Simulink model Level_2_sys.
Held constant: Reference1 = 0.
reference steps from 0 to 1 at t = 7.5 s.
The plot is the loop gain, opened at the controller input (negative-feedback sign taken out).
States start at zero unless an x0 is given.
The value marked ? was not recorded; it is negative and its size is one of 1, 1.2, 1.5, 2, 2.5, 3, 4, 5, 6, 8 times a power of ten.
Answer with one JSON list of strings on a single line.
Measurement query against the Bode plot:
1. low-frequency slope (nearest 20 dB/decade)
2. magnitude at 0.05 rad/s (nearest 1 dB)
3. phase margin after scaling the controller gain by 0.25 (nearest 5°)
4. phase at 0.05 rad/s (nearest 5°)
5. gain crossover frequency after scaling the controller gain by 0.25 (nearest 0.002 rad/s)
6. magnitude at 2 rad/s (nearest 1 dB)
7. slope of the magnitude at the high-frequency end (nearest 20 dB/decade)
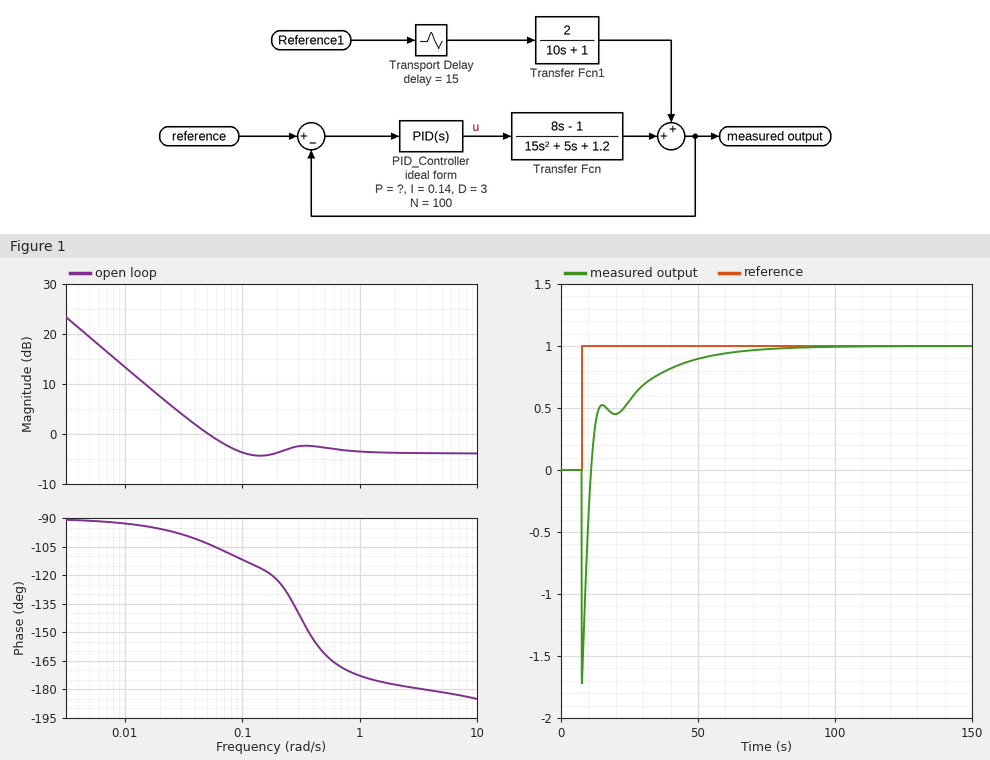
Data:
["-20 dB/decade", "0 dB", "85°", "-105°", "0.012 rad/s", "-4 dB", "0 dB/decade"]
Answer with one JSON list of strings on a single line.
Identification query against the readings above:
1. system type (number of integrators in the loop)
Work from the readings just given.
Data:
["1"]
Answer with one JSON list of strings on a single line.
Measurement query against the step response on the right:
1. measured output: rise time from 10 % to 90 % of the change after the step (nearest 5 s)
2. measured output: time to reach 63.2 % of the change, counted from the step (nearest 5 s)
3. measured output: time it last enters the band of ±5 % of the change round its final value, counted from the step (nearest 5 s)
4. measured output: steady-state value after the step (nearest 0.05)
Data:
["40 s", "20 s", "55 s", "1.00"]
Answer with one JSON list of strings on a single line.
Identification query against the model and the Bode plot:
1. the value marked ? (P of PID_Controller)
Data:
["-0.4"]
